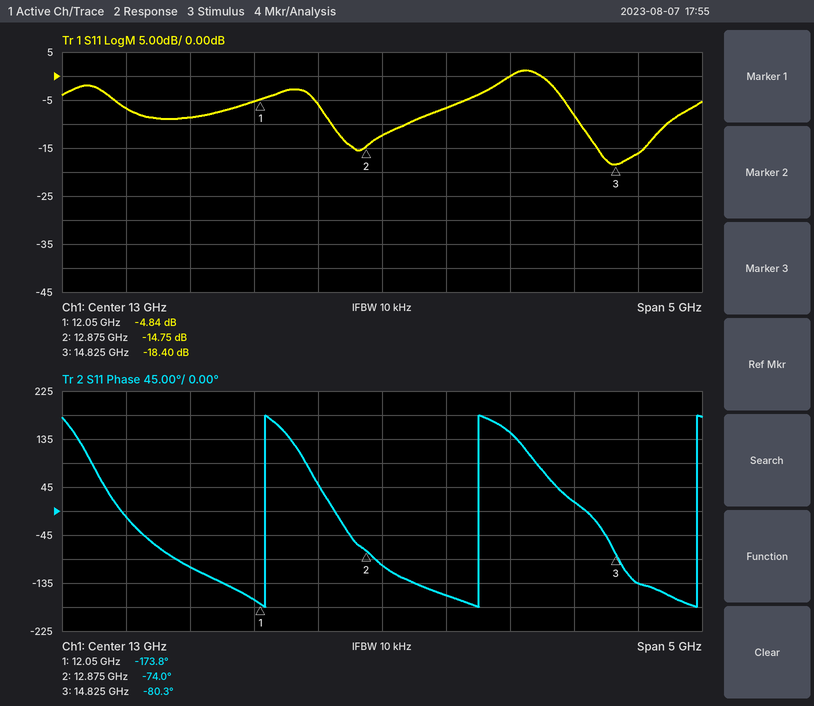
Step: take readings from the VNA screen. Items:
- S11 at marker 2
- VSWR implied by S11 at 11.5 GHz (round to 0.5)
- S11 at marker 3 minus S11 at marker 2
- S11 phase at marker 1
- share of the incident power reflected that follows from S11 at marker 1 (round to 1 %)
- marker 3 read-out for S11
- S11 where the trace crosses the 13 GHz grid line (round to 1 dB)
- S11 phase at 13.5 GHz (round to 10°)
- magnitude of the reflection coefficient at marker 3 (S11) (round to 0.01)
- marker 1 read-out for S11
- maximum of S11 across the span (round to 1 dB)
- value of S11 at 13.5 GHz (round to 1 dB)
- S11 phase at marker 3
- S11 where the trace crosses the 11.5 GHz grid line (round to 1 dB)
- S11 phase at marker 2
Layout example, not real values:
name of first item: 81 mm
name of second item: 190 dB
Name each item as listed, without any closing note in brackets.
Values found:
S11 at marker 2: -14.75 dB
VSWR implied by S11 at 11.5 GHz: 2.0
S11 at marker 3 minus S11 at marker 2: -3.65 dB
S11 phase at marker 1: -173.8°
share of the incident power reflected that follows from S11 at marker 1: 33 %
marker 3 read-out for S11: -18.40 dB
S11 where the trace crosses the 13 GHz grid line: -12 dB
S11 phase at 13.5 GHz: -160°
magnitude of the reflection coefficient at marker 3 (S11): 0.12
marker 1 read-out for S11: -4.84 dB
maximum of S11 across the span: 1 dB
value of S11 at 13.5 GHz: -7 dB
S11 phase at marker 3: -80.3°
S11 where the trace crosses the 11.5 GHz grid line: -9 dB
S11 phase at marker 2: -74.0°
